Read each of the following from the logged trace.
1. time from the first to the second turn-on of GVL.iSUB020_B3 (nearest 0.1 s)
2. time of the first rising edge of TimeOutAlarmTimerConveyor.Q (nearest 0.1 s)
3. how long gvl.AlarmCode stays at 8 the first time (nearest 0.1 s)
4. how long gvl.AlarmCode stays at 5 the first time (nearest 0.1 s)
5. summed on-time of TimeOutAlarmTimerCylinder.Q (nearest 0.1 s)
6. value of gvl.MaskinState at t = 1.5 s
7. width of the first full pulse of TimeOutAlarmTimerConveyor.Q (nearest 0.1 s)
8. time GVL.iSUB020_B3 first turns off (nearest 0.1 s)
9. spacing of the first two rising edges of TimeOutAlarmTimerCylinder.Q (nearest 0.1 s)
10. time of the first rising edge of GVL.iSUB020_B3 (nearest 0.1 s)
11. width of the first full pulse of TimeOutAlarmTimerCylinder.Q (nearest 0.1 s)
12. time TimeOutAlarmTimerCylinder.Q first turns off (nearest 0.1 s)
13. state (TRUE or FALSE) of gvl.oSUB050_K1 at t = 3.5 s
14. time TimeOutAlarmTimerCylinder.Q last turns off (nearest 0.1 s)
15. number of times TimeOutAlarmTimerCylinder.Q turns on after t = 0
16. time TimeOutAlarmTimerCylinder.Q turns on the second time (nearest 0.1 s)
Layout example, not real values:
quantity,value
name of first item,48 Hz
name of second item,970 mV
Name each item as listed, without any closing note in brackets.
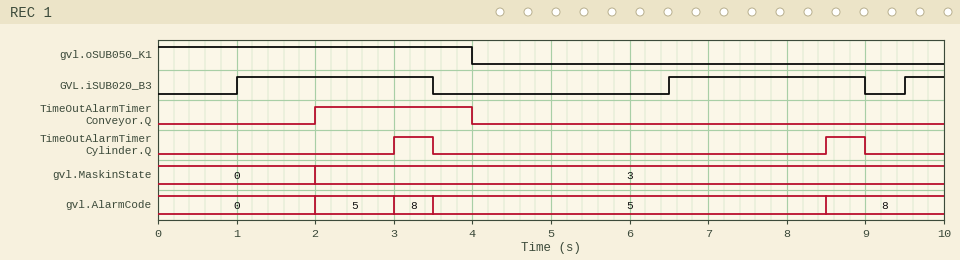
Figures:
quantity,value
time from the first to the second turn-on of GVL.iSUB020_B3,5.5 s
time of the first rising edge of TimeOutAlarmTimerConveyor.Q,2.0 s
how long gvl.AlarmCode stays at 8 the first time,0.5 s
how long gvl.AlarmCode stays at 5 the first time,1.0 s
summed on-time of TimeOutAlarmTimerCylinder.Q,1.0 s
value of gvl.MaskinState at t = 1.5 s,0
width of the first full pulse of TimeOutAlarmTimerConveyor.Q,2.0 s
time GVL.iSUB020_B3 first turns off,3.5 s
spacing of the first two rising edges of TimeOutAlarmTimerCylinder.Q,5.5 s
time of the first rising edge of GVL.iSUB020_B3,1.0 s
width of the first full pulse of TimeOutAlarmTimerCylinder.Q,0.5 s
time TimeOutAlarmTimerCylinder.Q first turns off,3.5 s
state (TRUE or FALSE) of gvl.oSUB050_K1 at t = 3.5 s,TRUE
time TimeOutAlarmTimerCylinder.Q last turns off,9.0 s
number of times TimeOutAlarmTimerCylinder.Q turns on after t = 0,2
time TimeOutAlarmTimerCylinder.Q turns on the second time,8.5 s
